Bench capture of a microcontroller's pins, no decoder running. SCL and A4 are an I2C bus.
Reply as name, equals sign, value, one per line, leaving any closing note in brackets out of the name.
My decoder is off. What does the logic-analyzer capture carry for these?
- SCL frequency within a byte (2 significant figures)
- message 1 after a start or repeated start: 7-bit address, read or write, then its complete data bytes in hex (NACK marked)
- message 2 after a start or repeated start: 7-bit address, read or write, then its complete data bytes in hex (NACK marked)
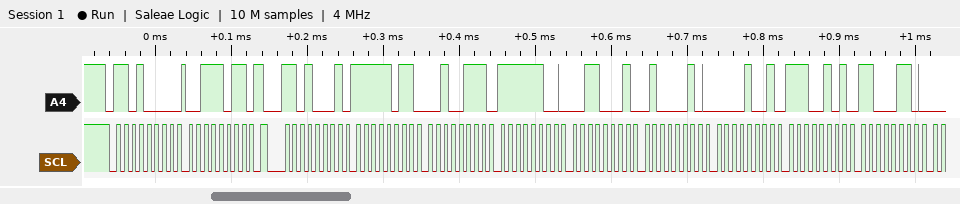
SCL frequency within a byte = 100 kHz
message 1 after a start or repeated start: 7-bit address, read or write, then its complete data bytes in hex = 0x68 write: 3B
message 2 after a start or repeated start: 7-bit address, read or write, then its complete data bytes in hex = 0x68 read: FB 27 FC 31 42 09 E5 C6
